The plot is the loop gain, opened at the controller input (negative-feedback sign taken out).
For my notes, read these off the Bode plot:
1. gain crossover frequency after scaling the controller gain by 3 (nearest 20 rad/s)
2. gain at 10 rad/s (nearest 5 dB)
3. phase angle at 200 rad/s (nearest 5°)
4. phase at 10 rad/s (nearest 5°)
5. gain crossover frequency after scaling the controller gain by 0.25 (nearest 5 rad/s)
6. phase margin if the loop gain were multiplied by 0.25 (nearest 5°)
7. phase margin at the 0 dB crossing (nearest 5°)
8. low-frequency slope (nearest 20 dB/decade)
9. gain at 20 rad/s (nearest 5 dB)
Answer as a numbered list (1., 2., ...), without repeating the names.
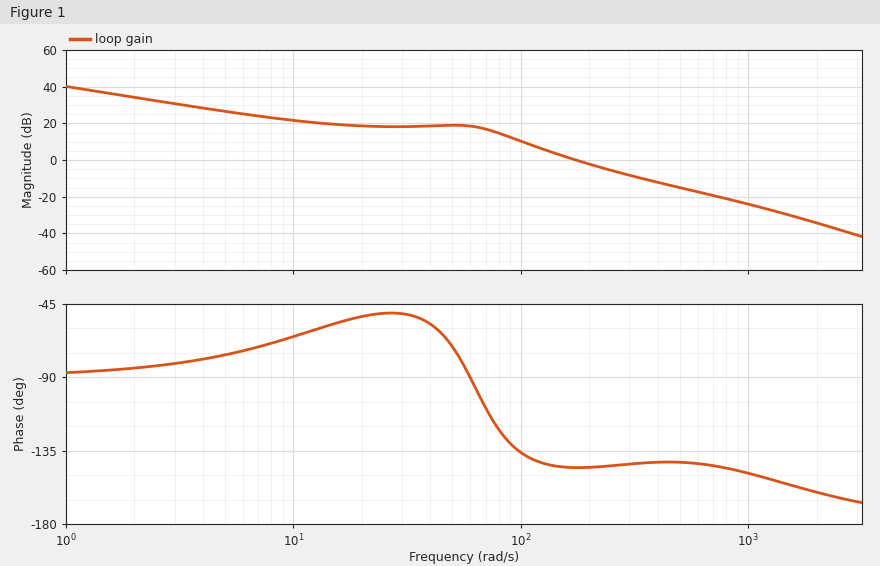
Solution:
1. 320 rad/s
2. 20 dB
3. -145°
4. -65°
5. 90 rad/s
6. 50°
7. 35°
8. -20 dB/decade
9. 20 dB
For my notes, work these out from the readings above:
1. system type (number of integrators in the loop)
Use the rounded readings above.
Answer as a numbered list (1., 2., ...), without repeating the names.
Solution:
1. 1
